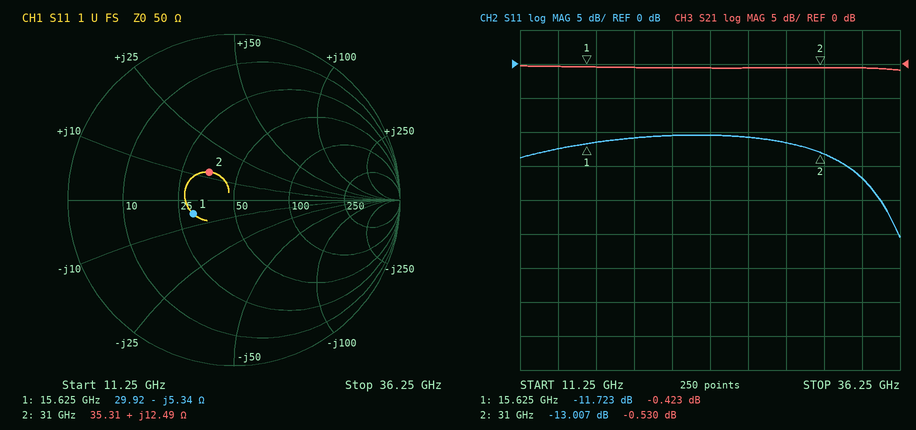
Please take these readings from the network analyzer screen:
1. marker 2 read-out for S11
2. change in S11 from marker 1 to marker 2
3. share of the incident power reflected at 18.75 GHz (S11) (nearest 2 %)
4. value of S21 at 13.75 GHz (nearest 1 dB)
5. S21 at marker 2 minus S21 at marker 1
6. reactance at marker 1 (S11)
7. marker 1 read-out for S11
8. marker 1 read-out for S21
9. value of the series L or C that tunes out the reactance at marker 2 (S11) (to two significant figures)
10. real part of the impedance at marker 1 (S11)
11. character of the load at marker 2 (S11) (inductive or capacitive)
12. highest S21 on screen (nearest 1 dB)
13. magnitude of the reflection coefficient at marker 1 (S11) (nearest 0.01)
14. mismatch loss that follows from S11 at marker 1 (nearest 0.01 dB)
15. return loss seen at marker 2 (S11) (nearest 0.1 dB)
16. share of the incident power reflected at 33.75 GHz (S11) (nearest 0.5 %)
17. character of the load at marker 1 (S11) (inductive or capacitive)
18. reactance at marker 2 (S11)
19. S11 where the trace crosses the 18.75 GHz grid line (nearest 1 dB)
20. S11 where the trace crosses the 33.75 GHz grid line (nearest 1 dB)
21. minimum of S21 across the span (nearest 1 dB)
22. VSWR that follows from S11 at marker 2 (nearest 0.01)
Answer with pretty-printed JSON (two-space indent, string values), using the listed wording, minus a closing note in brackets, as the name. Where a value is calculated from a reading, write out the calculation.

{
  "marker 2 read-out for S11": "-13.007 dB",
  "change in S11 from marker 1 to marker 2": "-13.007 − (-11.723) = -1.284 dB",
  "share of the incident power reflected at 18.75 GHz (S11)": "10^(-11/10) ≈ 8 %",
  "value of S21 at 13.75 GHz": "0 dB",
  "S21 at marker 2 minus S21 at marker 1": "-0.53 − (-0.423) = -0.107 dB",
  "reactance at marker 1": "-5.34 Ω",
  "marker 1 read-out for S11": "-11.723 dB",
  "marker 1 read-out for S21": "-0.423 dB",
  "value of the series L or C that tunes out the reactance at marker 2 (S11)": "C = 1/(2π × 31 GHz × 12.49 Ω) ≈ 411 fF, so 410 fF to two significant figures",
  "real part of the impedance at marker 1": "29.92 Ω",
  "character of the load at marker 2 (S11)": "inductive",
  "highest S21 on screen": "0 dB",
  "magnitude of the reflection coefficient at marker 1 (S11)": "0.26",
  "mismatch loss that follows from S11 at marker 1": "−10 log10(1 − 10^(-11.723/10)) ≈ 0.30 dB",
  "return loss seen at marker 2 (S11)": "13.0 dB",
  "share of the incident power reflected at 33.75 GHz (S11)": "10^(-17/10) ≈ 2.0 %",
  "character of the load at marker 1 (S11)": "capacitive",
  "reactance at marker 2": "+12.49 Ω",
  "S11 where the trace crosses the 18.75 GHz grid line": "-11 dB",
  "S11 where the trace crosses the 33.75 GHz grid line": "-17 dB",
  "minimum of S21 across the span": "-1 dB",
  "VSWR that follows from S11 at marker 2": "(1 + 0.2237)/(1 − 0.2237) ≈ 1.58"
}
